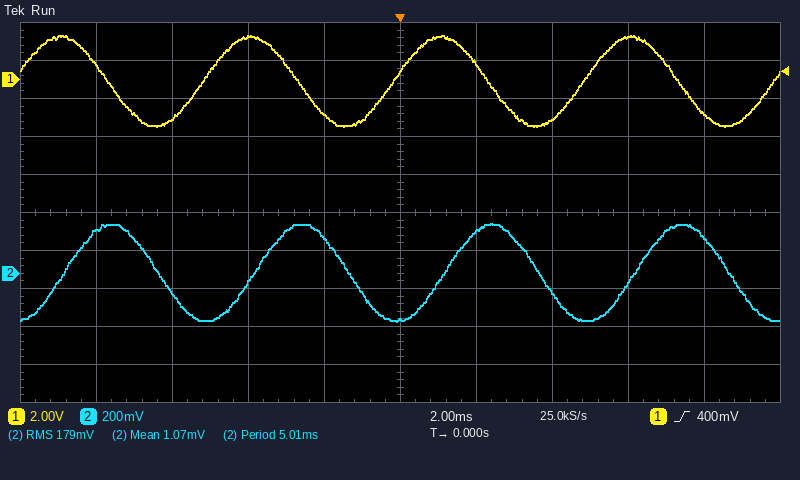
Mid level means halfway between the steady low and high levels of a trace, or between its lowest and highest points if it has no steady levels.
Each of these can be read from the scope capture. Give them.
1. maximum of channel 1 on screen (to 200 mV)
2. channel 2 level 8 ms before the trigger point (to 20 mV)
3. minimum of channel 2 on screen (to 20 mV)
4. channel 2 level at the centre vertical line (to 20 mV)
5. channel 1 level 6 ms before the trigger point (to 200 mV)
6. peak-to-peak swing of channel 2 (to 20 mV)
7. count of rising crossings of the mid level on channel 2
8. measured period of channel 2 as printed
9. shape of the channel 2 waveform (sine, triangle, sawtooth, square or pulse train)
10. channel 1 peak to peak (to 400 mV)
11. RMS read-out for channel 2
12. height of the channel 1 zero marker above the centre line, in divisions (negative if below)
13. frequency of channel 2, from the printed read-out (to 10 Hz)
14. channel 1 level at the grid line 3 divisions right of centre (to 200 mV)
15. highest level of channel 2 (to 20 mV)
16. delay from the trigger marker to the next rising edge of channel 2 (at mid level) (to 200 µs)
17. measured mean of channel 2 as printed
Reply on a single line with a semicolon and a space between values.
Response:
2.4 V; 220 mV; -260 mV; -240 mV; -2.0 V; 520 mV; 4; 5.01 ms; sine; 4.8 V; 179 mV; +3.5 div; 200 Hz; 2.2 V; 260 mV; 1.2 ms; 1.07 mV
